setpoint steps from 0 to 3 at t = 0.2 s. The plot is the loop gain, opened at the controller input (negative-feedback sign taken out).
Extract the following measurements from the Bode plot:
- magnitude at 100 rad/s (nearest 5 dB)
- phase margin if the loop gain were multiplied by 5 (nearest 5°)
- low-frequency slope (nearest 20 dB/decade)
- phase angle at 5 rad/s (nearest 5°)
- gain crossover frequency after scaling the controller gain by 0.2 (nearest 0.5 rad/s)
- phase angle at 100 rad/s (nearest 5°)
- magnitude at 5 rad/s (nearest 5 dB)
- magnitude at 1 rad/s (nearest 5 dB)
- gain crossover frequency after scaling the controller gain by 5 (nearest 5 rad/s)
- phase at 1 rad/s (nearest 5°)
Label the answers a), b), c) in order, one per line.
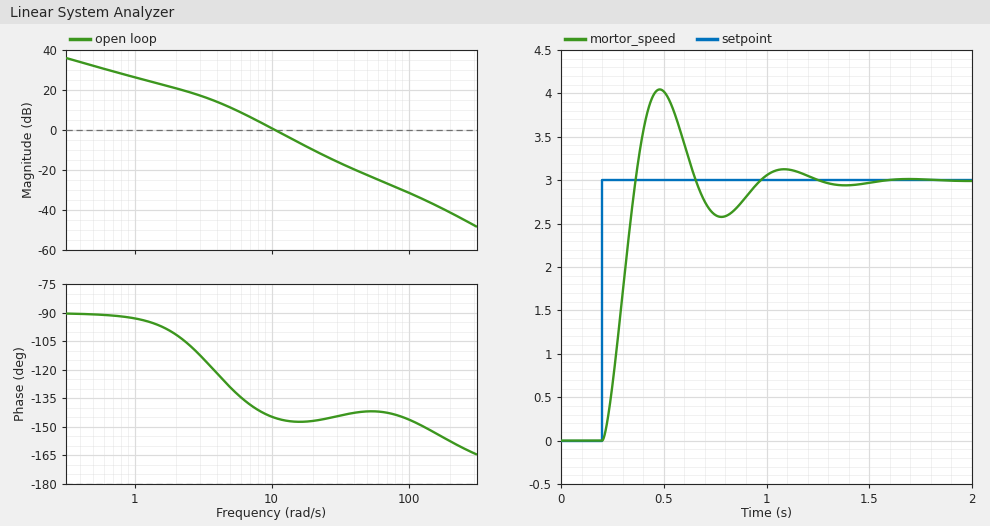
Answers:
a) -30 dB
b) 35°
c) -20 dB/decade
d) -130°
e) 4.0 rad/s
f) -145°
g) 10 dB
h) 25 dB
i) 25 rad/s
j) -95°
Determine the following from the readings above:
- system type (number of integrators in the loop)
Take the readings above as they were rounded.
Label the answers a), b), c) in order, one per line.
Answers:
a) 1
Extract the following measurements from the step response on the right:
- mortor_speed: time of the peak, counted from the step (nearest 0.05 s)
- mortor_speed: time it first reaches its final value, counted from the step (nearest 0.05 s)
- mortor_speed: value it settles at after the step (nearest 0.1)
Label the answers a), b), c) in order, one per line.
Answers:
a) 0.30 s
b) 0.15 s
c) 3.0
